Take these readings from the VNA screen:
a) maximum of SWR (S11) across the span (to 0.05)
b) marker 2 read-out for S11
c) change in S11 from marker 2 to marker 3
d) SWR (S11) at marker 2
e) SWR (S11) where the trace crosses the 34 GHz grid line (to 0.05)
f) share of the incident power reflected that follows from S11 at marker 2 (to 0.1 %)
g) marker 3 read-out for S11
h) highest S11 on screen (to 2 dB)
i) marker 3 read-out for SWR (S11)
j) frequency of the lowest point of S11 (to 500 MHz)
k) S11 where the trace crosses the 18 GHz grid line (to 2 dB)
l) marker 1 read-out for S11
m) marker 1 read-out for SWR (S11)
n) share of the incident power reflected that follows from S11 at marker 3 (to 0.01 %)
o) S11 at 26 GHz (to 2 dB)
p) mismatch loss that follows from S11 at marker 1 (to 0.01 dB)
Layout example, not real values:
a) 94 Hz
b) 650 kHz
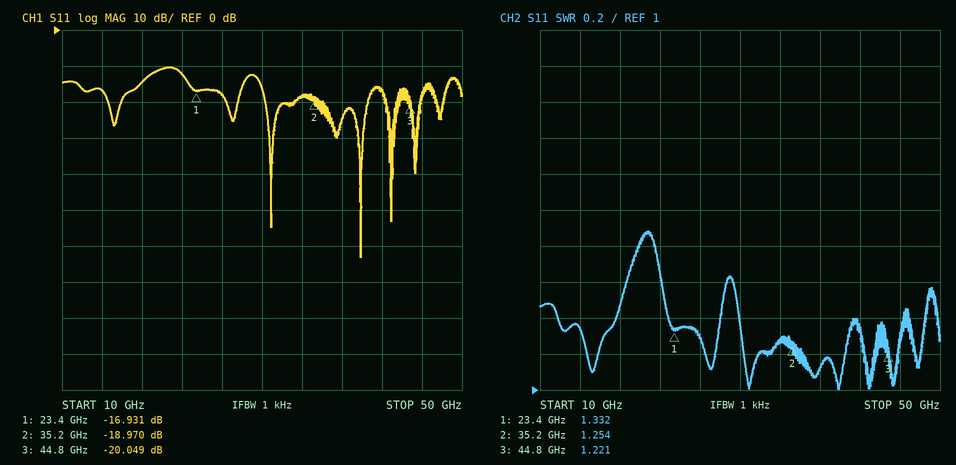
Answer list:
a) 1.90
b) -18.970 dB
c) -1.079 dB
d) 1.254
e) 1.25
f) 1.3 %
g) -20.049 dB
h) -10 dB
i) 1.221
j) 40.0 GHz
k) -14 dB
l) -16.931 dB
m) 1.332
n) 0.99 %
o) -18 dB
p) 0.09 dB
